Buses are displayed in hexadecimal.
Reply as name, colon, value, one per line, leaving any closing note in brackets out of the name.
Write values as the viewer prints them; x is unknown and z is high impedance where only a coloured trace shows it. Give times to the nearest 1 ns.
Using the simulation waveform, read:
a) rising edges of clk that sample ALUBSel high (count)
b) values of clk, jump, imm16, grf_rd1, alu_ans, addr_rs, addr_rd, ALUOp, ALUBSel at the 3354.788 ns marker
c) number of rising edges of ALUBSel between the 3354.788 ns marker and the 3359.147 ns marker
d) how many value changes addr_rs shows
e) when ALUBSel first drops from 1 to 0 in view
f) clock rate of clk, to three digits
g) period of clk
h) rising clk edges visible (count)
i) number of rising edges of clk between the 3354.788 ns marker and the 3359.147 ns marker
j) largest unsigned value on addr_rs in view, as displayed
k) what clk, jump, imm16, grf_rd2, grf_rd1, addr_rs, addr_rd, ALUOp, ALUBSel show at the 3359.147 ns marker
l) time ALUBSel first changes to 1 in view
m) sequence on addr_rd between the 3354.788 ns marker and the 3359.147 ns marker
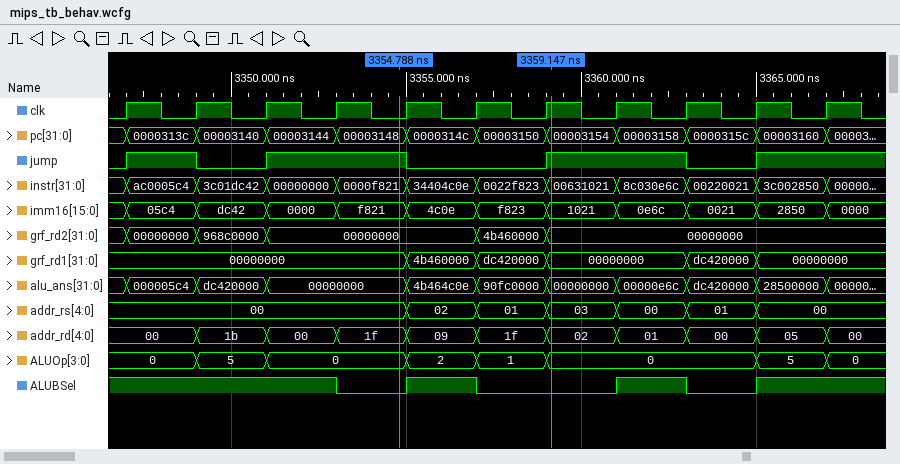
rising edges of clk that sample ALUBSel high: 7
values of clk, jump, imm16, grf_rd1, alu_ans, addr_rs, addr_rd, ALUOp, ALUBSel at the 3354.788 ns marker: clk=0, jump=1, imm16=f821, grf_rd1=00000000, alu_ans=00000000, addr_rs=00, addr_rd=1f, ALUOp=0, ALUBSel=0
number of rising edges of ALUBSel between the 3354.788 ns marker and the 3359.147 ns marker: 1
how many value changes addr_rs shows: 6
when ALUBSel first drops from 1 to 0 in view: 3353 ns
clock rate of clk, to three digits: 500 MHz
period of clk: 2 ns
rising clk edges visible: 11
number of rising edges of clk between the 3354.788 ns marker and the 3359.147 ns marker: 3
largest unsigned value on addr_rs in view, as displayed: 03
what clk, jump, imm16, grf_rd2, grf_rd1, addr_rs, addr_rd, ALUOp, ALUBSel show at the 3359.147 ns marker: clk=1, jump=1, imm16=1021, grf_rd2=00000000, grf_rd1=00000000, addr_rs=03, addr_rd=02, ALUOp=0, ALUBSel=0
time ALUBSel first changes to 1 in view: 3355 ns
sequence on addr_rd between the 3354.788 ns marker and the 3359.147 ns marker: 1f, 09, 1f, 02
